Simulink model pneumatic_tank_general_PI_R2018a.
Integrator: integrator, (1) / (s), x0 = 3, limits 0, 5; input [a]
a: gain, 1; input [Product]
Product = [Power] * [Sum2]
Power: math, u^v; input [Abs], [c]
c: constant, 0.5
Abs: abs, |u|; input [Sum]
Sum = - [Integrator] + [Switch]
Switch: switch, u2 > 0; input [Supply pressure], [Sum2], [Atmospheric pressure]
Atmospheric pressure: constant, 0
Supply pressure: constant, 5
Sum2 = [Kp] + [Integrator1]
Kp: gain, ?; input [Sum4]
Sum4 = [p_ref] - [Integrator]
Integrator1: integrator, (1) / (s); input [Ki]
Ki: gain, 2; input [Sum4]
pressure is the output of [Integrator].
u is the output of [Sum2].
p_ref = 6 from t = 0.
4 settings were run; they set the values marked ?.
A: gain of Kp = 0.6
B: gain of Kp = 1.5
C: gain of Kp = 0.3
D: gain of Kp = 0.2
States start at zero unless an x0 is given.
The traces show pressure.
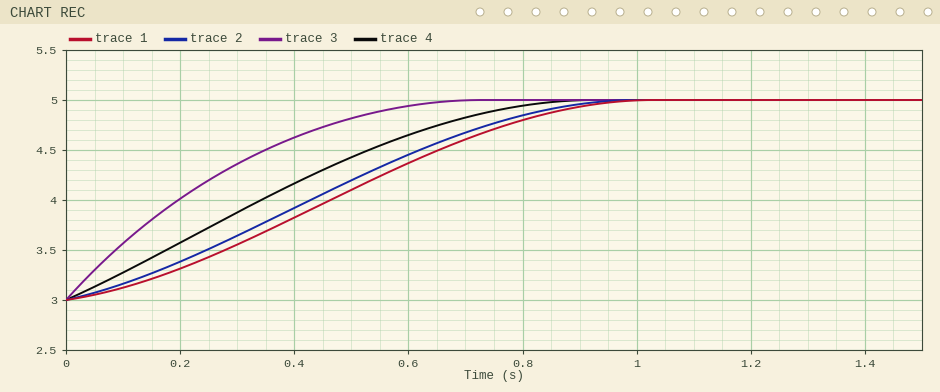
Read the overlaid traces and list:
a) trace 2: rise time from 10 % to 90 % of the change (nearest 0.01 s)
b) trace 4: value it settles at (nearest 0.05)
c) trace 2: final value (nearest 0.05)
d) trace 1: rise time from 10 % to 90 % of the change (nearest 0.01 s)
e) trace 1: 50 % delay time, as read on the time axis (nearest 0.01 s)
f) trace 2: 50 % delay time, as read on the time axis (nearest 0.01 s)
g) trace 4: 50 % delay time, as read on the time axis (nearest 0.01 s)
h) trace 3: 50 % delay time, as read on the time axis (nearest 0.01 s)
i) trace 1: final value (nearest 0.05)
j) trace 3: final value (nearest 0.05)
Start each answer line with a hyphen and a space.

- 0.65 s
- 5.00
- 5.00
- 0.66 s
- 0.46 s
- 0.43 s
- 0.34 s
- 0.20 s
- 5.00
- 5.00
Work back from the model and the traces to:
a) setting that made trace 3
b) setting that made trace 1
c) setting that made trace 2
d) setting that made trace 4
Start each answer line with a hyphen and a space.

- B
- D
- C
- A
